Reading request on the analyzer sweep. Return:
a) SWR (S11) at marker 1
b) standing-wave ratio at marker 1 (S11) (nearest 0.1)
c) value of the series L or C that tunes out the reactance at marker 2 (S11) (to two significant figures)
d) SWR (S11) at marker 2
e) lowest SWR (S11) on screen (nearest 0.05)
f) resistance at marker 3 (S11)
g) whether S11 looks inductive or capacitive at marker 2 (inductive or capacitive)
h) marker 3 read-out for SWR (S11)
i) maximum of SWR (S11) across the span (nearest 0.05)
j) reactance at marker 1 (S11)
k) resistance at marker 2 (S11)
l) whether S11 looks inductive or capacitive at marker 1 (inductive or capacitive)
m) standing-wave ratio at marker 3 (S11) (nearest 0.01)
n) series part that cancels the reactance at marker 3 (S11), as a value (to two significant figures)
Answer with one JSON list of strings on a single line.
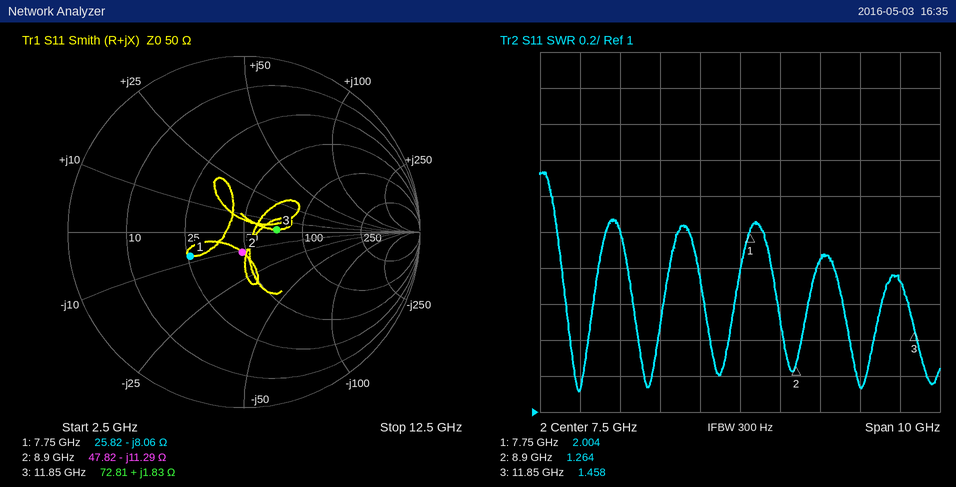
["2.004", "2.0", "200 pH", "1.264", "1.10", "72.81 Ω", "capacitive", "1.458", "2.35", "-8.06 Ω", "47.82 Ω", "capacitive", "1.46", "7.3 pF"]
